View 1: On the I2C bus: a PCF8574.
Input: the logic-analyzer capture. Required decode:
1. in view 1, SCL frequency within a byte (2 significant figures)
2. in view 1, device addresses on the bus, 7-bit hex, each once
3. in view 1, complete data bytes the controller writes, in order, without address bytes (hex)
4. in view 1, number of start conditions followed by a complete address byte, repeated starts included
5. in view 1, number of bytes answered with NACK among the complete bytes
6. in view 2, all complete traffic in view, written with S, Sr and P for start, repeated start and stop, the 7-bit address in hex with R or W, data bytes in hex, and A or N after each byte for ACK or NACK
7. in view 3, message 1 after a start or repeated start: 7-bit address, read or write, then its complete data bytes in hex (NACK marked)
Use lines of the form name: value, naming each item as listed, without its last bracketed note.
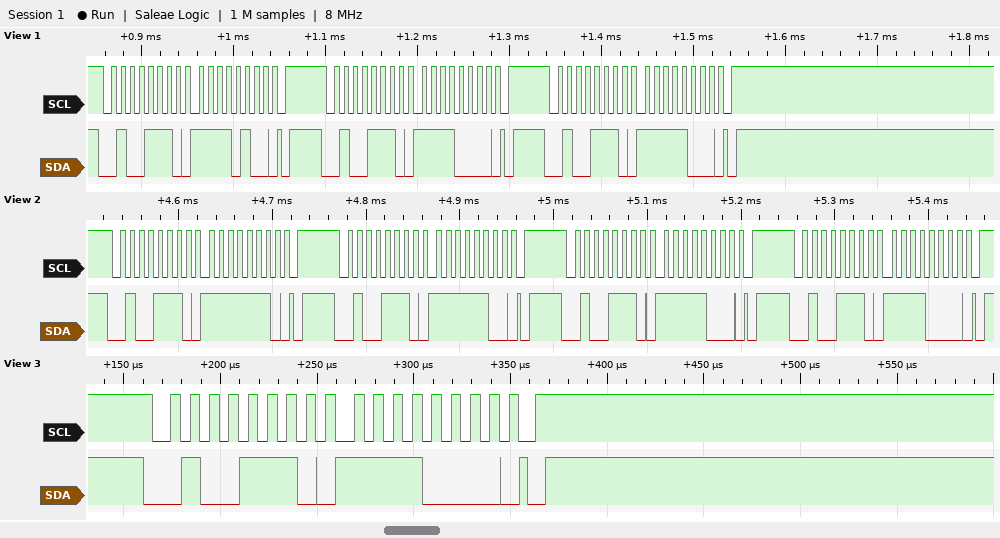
in view 1, SCL frequency within a byte: 100 kHz
in view 1, device addresses on the bus, 7-bit hex, each once: 0x27
in view 1, complete data bytes the controller writes, in order, without address bytes: F4 F0 F8
in view 1, number of start conditions followed by a complete address byte, repeated starts included: 3
in view 1, number of bytes answered with NACK among the complete bytes: 0
in view 2, all complete traffic in view, written with S, Sr and P for start, repeated start and stop, the 7-bit address in hex with R or W, data bytes in hex, and A or N after each byte for ACK or NACK: S 27W A FE A P S 27W A FC A P S 27W A F8 A P S 27W A F0 A P
in view 3, message 1 after a start or repeated start: 7-bit address, read or write, then its complete data bytes in hex: 0x27 write: F0
